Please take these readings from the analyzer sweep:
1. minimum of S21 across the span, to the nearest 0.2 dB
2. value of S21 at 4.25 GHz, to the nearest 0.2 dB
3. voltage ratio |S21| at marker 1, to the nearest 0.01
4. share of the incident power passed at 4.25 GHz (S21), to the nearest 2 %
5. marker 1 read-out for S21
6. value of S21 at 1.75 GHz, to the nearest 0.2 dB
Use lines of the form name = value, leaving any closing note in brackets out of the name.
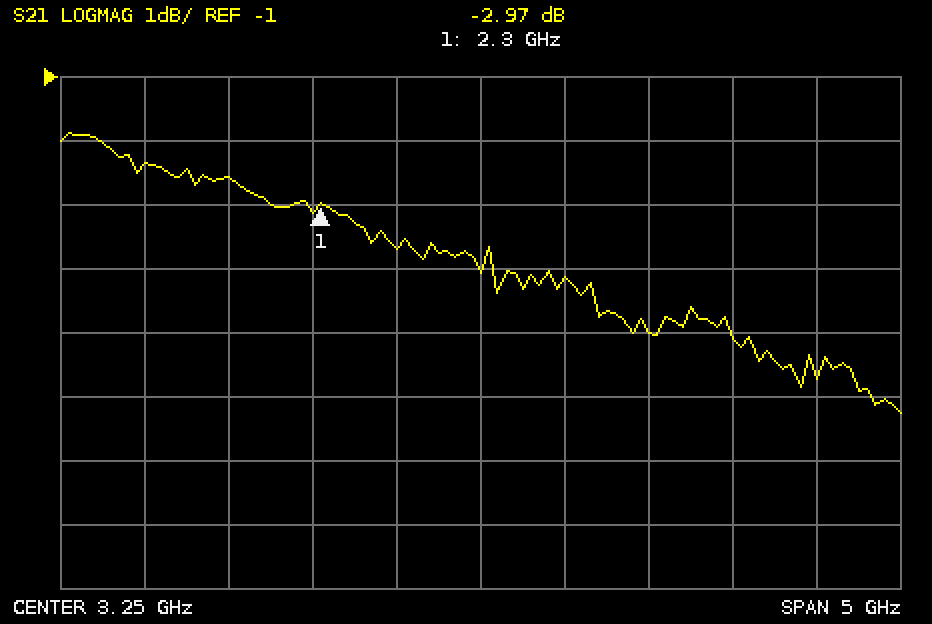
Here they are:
minimum of S21 across the span, to the nearest 0.2 dB = -6.2 dB
value of S21 at 4.25 GHz, to the nearest 0.2 dB = -5.0 dB
voltage ratio |S21| at marker 1, to the nearest 0.01 = 0.71
share of the incident power passed at 4.25 GHz (S21), to the nearest 2 % = 32 %
marker 1 read-out for S21 = -2.97 dB
value of S21 at 1.75 GHz, to the nearest 0.2 dB = -2.6 dB
